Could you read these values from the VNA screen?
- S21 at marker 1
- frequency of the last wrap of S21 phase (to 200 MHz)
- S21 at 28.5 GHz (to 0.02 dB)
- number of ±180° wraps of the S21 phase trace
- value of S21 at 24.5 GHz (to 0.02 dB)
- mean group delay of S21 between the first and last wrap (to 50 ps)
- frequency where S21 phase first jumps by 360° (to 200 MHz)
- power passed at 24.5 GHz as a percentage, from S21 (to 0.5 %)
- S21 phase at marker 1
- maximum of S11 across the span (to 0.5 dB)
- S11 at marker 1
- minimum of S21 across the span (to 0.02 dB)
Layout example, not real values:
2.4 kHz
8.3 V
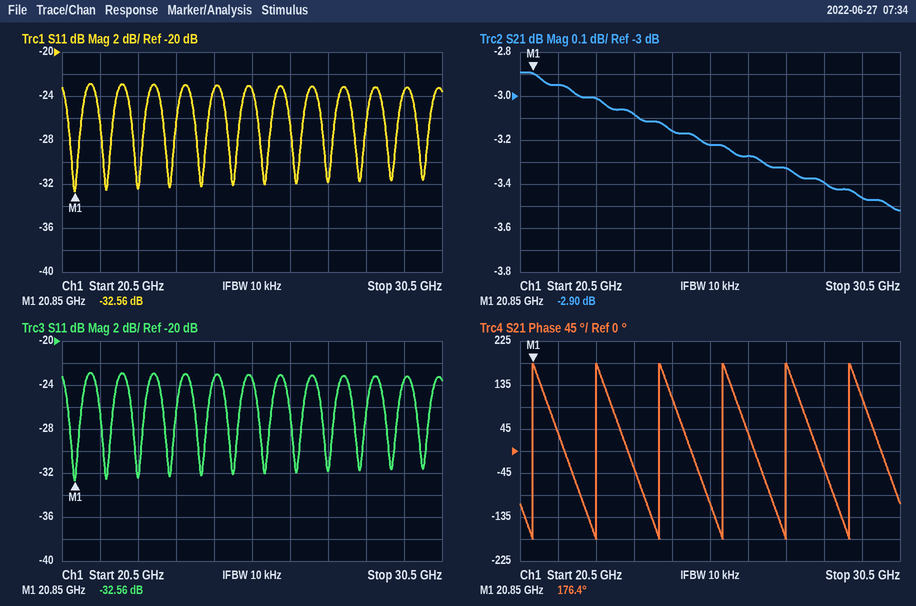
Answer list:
-2.90 dB
29.2 GHz
-3.40 dB
6
-3.16 dB
600 ps
20.8 GHz
48.5 %
176.4°
-23.0 dB
-32.56 dB
-3.52 dB
